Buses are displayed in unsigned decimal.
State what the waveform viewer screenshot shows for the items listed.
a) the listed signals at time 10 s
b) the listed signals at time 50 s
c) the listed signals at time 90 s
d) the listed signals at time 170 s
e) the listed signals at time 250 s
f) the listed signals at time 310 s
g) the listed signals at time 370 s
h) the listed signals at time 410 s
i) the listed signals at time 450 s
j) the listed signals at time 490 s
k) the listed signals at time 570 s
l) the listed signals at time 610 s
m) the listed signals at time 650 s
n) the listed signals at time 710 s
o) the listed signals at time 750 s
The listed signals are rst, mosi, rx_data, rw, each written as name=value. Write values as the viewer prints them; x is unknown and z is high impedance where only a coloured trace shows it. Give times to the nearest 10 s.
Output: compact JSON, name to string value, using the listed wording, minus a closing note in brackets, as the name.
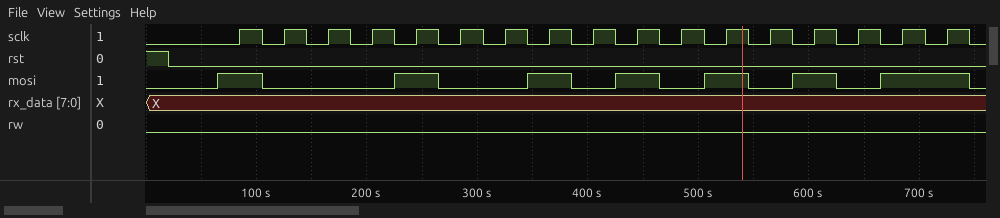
{"the listed signals at time 10 s": "rst=1, mosi=0, rx_data=X, rw=0", "the listed signals at time 50 s": "rst=0, mosi=0, rx_data=X, rw=0", "the listed signals at time 90 s": "rst=0, mosi=1, rx_data=X, rw=0", "the listed signals at time 170 s": "rst=0, mosi=0, rx_data=X, rw=0", "the listed signals at time 250 s": "rst=0, mosi=1, rx_data=X, rw=0", "the listed signals at time 310 s": "rst=0, mosi=0, rx_data=X, rw=0", "the listed signals at time 370 s": "rst=0, mosi=1, rx_data=X, rw=0", "the listed signals at time 410 s": "rst=0, mosi=0, rx_data=X, rw=0", "the listed signals at time 450 s": "rst=0, mosi=1, rx_data=X, rw=0", "the listed signals at time 490 s": "rst=0, mosi=0, rx_data=X, rw=0", "the listed signals at time 570 s": "rst=0, mosi=0, rx_data=X, rw=0", "the listed signals at time 610 s": "rst=0, mosi=1, rx_data=X, rw=0", "the listed signals at time 650 s": "rst=0, mosi=0, rx_data=X, rw=0", "the listed signals at time 710 s": "rst=0, mosi=1, rx_data=X, rw=0", "the listed signals at time 750 s": "rst=0, mosi=0, rx_data=X, rw=0"}
